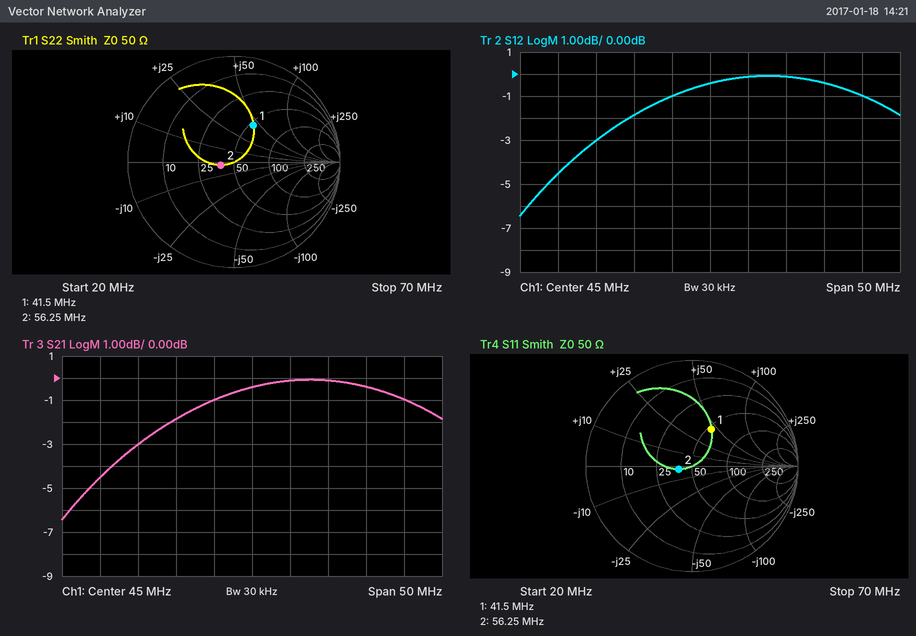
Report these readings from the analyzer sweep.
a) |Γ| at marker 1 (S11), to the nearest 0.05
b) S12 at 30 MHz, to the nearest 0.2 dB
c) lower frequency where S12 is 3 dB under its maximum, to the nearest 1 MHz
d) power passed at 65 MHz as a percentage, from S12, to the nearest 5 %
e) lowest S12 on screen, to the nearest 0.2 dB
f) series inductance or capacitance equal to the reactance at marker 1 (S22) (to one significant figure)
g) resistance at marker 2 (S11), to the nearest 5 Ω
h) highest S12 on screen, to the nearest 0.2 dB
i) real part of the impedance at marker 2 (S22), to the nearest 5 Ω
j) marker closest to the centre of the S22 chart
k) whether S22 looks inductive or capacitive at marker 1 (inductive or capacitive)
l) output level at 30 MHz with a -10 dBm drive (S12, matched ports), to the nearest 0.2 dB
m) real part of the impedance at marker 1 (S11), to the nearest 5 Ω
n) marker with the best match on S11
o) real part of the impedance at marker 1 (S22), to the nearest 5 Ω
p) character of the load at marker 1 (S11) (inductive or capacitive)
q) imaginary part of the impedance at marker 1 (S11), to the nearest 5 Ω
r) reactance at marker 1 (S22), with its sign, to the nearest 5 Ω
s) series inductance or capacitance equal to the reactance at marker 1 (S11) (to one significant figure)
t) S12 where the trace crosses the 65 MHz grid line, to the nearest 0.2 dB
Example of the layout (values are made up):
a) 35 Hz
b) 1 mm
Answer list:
a) 0.40
b) -3.0 dB
c) 30 MHz
d) 80 %
e) -6.4 dB
f) 200 nH
g) 40 Ω
h) 0.0 dB
i) 40 Ω
j) marker 2
k) inductive
l) -13.0 dBm
m) 55 Ω
n) marker 2
o) 55 Ω
p) inductive
q) +45 Ω
r) +45 Ω
s) 200 nH
t) -1.0 dB
